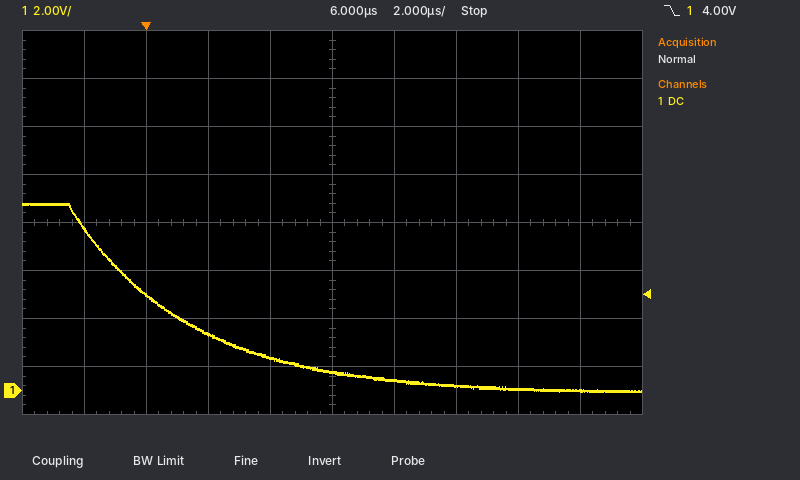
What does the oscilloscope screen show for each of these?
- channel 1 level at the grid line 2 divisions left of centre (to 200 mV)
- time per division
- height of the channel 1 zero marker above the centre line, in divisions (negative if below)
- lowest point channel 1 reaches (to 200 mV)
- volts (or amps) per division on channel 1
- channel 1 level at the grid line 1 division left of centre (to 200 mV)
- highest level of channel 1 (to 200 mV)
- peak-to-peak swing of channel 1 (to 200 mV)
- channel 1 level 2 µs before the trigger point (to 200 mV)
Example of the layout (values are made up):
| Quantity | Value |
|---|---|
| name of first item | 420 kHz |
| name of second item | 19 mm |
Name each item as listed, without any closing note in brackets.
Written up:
| Quantity | Value |
|---|---|
| channel 1 level at the grid line 2 divisions left of centre | 2.4 V |
| time per division | 2 µs |
| height of the channel 1 zero marker above the centre line, in divisions | -3.5 div |
| lowest point channel 1 reaches | 0.0 V |
| volts (or amps) per division on channel 1 | 2 V |
| channel 1 level at the grid line 1 division left of centre | 1.4 V |
| highest level of channel 1 | 7.8 V |
| peak-to-peak swing of channel 1 | 7.8 V |
| channel 1 level 2 µs before the trigger point | 6.8 V |
